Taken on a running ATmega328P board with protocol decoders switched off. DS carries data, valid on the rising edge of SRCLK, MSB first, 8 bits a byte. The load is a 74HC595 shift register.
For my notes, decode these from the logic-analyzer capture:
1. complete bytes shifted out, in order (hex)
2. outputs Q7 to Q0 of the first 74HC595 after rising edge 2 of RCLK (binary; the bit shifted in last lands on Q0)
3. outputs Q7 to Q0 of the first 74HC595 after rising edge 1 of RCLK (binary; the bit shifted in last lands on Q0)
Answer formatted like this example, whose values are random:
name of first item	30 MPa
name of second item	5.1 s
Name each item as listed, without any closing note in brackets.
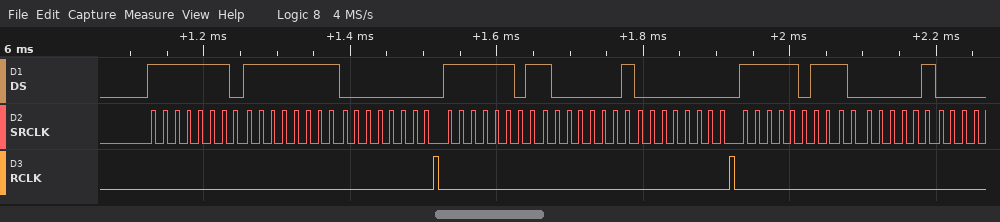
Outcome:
complete bytes shifted out, in order	0xFE 0xFF 0x00 0xFD 0x81 0x00 0xFB 0x81
outputs Q7 to Q0 of the first 74HC595 after rising edge 2 of RCLK	00000000
outputs Q7 to Q0 of the first 74HC595 after rising edge 1 of RCLK	00000000
